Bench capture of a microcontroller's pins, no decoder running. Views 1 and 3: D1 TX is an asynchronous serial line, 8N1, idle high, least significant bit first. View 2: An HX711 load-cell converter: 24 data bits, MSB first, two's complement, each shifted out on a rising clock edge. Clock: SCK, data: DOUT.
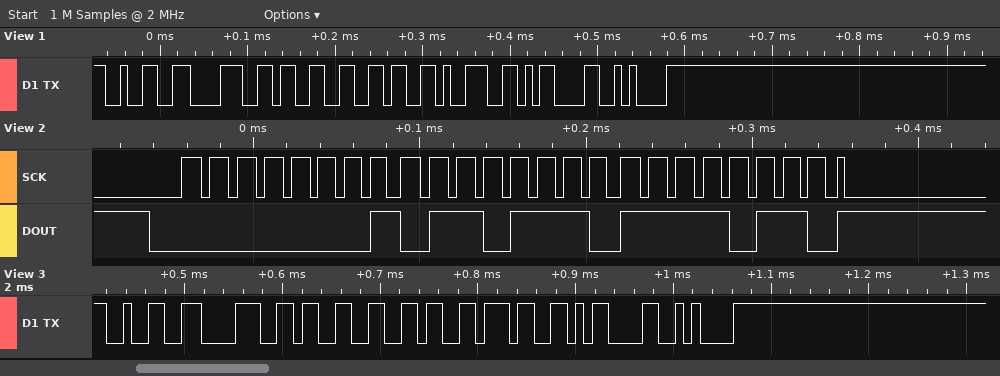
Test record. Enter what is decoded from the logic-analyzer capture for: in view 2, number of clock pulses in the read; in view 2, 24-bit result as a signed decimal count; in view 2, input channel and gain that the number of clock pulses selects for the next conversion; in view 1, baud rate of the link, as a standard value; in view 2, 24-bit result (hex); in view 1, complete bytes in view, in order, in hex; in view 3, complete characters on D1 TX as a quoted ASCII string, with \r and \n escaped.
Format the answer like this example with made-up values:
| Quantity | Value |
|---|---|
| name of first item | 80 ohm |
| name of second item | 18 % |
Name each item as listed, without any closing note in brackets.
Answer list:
| Quantity | Value |
|---|---|
| in view 2, number of clock pulses in the read | 25 |
| in view 2, 24-bit result as a signed decimal count | 93942 |
| in view 2, input channel and gain that the number of clock pulses selects for the next conversion | channel A, gain 128 |
| in view 1, baud rate of the link, as a standard value | 115200 baud |
| in view 2, 24-bit result | 0x016EF6 |
| in view 1, complete bytes in view, in order, in hex | 0x32 0x38 0x33 0x36 0x39 0x0D 0x0A |
| in view 3, complete characters on D1 TX as a quoted ASCII string, with \r and \n escaped | "28367\r\n" |
